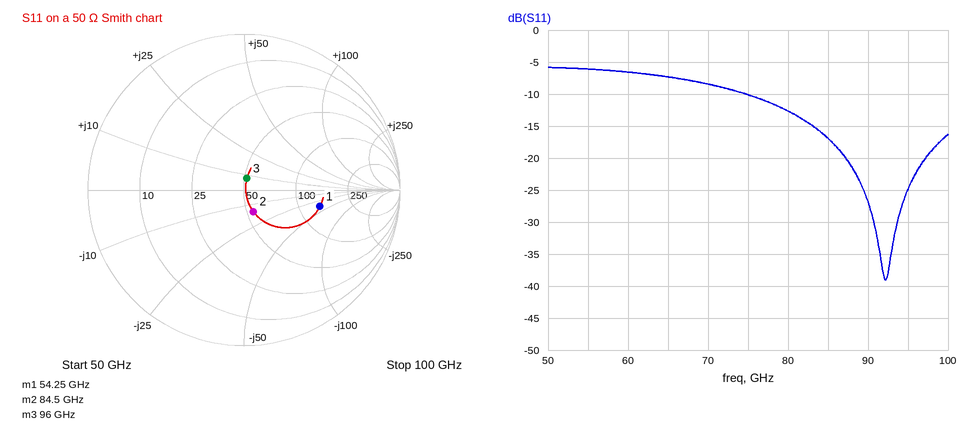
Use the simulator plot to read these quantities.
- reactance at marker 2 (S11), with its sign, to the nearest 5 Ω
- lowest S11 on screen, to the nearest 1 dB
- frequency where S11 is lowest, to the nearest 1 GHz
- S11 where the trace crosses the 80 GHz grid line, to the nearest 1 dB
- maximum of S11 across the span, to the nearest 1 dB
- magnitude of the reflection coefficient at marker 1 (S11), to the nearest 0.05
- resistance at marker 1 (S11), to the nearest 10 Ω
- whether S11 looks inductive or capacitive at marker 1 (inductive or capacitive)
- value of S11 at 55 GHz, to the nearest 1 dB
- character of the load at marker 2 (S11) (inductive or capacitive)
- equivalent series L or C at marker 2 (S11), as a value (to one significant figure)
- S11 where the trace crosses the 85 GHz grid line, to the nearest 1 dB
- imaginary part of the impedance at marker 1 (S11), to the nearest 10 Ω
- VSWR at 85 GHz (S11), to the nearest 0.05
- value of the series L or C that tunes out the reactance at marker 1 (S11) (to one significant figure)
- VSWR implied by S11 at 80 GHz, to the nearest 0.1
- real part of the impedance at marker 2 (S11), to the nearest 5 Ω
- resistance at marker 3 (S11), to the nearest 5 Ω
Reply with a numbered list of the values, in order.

1. -15 Ω
2. -39 dB
3. 92 GHz
4. -13 dB
5. -6 dB
6. 0.50
7. 140 Ω
8. capacitive
9. -6 dB
10. capacitive
11. 100 fF
12. -17 dB
13. -40 Ω
14. 1.35
15. 100 pH
16. 1.6
17. 55 Ω
18. 50 Ω
